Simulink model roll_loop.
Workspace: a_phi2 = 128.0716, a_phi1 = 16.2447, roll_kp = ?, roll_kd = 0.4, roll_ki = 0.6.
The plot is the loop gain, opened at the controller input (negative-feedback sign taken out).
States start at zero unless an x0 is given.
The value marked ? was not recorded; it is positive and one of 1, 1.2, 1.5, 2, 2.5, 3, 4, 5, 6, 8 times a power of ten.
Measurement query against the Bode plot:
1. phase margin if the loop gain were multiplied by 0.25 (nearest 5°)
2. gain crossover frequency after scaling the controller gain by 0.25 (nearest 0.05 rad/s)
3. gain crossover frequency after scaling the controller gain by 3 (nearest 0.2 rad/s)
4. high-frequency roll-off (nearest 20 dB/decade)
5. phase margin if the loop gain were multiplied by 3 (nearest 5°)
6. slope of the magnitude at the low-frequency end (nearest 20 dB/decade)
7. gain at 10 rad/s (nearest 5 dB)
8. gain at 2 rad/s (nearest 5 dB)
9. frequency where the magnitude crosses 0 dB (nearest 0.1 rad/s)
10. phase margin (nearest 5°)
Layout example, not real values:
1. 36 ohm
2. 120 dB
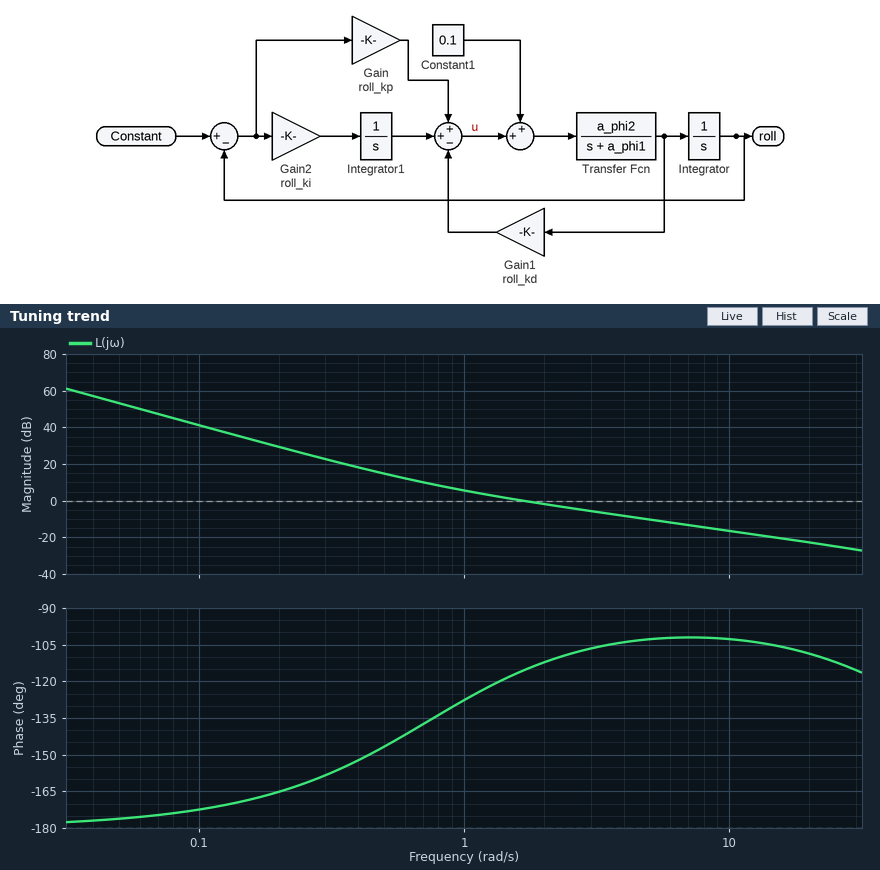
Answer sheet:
1. 40°
2. 0.60 rad/s
3. 4.6 rad/s
4. -20 dB/decade
5. 75°
6. -40 dB/decade
7. -15 dB
8. 0 dB
9. 1.7 rad/s
10. 65°
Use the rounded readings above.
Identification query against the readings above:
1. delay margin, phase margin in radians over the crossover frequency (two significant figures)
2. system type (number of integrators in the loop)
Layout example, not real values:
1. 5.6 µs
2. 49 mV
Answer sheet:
1. 0.67 s
2. 2
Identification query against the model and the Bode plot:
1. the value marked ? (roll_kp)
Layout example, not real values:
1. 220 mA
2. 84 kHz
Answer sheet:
1. 0.8
